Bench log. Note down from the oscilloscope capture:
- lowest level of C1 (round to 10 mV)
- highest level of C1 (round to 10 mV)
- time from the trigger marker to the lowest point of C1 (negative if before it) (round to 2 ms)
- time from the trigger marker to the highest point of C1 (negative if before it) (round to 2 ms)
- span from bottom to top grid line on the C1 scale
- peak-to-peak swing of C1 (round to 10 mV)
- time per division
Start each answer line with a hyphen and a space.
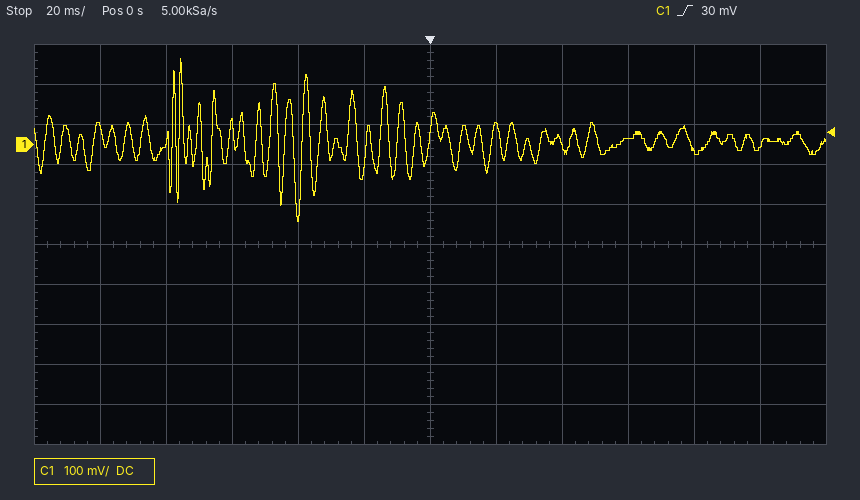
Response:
- -190 mV
- 220 mV
- -40 ms
- -76 ms
- 1 V
- 410 mV
- 20 ms
